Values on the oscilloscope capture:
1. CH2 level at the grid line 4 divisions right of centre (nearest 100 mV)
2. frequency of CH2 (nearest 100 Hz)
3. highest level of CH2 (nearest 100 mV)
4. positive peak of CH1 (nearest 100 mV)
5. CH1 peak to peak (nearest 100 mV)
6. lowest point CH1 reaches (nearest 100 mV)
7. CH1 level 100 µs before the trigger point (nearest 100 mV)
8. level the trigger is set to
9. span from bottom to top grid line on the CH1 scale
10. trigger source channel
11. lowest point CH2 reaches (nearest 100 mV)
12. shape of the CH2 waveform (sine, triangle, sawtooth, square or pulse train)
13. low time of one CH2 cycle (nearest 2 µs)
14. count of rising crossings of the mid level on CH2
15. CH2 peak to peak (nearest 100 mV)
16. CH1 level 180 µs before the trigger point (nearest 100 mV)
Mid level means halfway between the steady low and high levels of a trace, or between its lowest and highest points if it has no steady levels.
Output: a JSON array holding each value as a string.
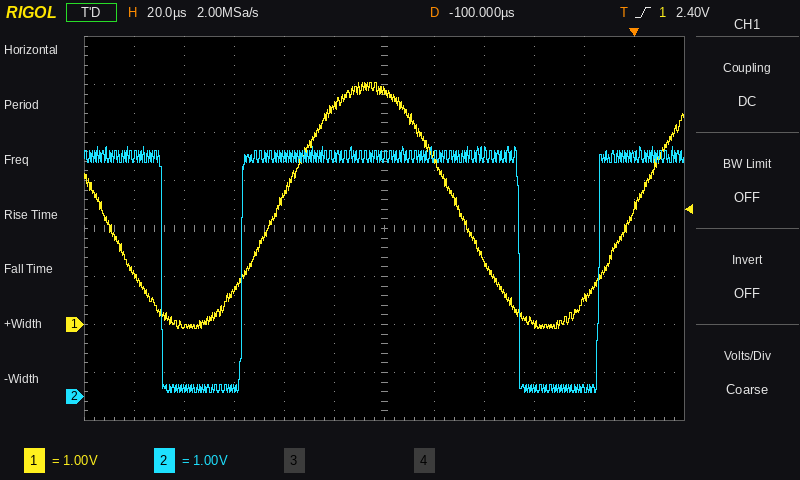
["200 mV", "7.0 kHz", "5.2 V", "5.0 V", "5.1 V", "-100 mV", "4.9 V", "2.40 V", "8 V", "CH1", "100 mV", "pulse train", "32 µs", "2", "5.1 V", "0.0 V"]
